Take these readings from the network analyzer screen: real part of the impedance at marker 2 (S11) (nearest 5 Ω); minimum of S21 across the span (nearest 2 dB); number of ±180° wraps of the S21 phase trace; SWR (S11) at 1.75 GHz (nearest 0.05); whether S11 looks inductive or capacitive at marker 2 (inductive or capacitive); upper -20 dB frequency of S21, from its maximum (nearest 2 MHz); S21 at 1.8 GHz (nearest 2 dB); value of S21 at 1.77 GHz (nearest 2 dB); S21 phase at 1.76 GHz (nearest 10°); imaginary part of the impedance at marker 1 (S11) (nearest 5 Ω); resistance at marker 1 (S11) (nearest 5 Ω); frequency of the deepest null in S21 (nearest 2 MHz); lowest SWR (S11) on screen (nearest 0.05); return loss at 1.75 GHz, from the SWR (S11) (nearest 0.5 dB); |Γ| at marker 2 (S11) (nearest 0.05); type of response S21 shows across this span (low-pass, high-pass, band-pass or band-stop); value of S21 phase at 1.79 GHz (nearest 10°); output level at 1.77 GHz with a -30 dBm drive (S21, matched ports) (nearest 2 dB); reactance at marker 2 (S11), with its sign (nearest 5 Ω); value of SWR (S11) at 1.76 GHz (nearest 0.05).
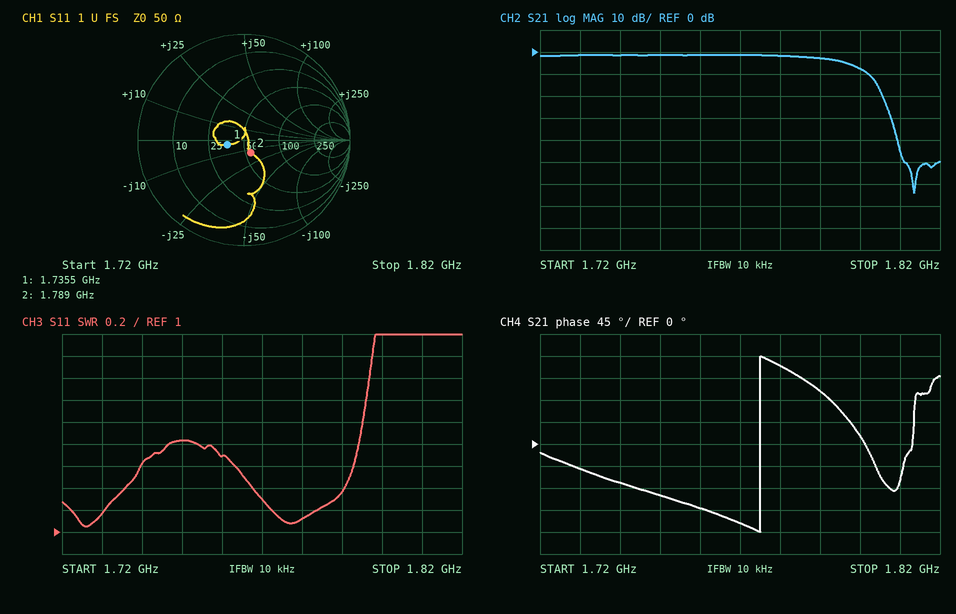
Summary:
55 Ω
-64 dB
1
1.85
capacitive
1.806 GHz
-8 dB
-2 dB
-130°
-5 Ω
35 Ω
1.814 GHz
1.05
10.5 dB
0.15
low-pass
110°
-32 dBm
-15 Ω
1.70
